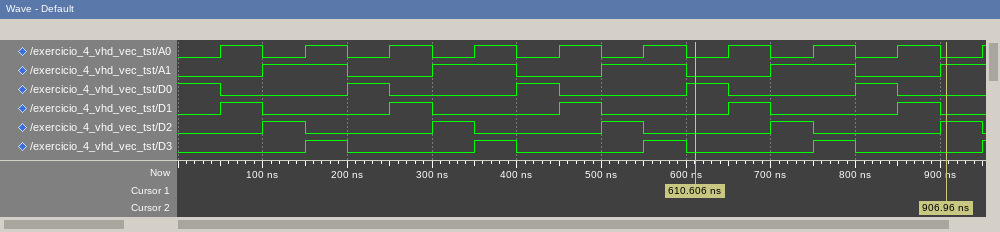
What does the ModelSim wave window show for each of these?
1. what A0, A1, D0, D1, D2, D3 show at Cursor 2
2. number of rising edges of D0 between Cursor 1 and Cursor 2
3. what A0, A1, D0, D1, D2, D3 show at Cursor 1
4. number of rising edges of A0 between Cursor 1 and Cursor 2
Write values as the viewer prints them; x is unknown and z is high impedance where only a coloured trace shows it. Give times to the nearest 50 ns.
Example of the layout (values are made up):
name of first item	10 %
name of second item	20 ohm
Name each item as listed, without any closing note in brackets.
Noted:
what A0, A1, D0, D1, D2, D3 show at Cursor 2	A0=0, A1=1, D0=0, D1=0, D2=1, D3=0
number of rising edges of D0 between Cursor 1 and Cursor 2	1
what A0, A1, D0, D1, D2, D3 show at Cursor 1	A0=0, A1=0, D0=1, D1=0, D2=0, D3=0
number of rising edges of A0 between Cursor 1 and Cursor 2	3
